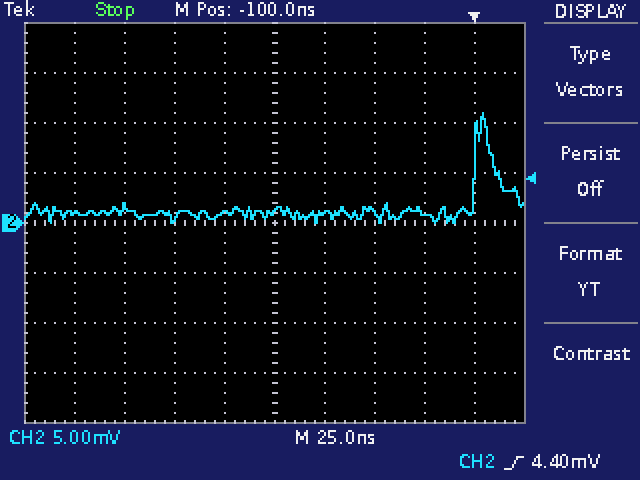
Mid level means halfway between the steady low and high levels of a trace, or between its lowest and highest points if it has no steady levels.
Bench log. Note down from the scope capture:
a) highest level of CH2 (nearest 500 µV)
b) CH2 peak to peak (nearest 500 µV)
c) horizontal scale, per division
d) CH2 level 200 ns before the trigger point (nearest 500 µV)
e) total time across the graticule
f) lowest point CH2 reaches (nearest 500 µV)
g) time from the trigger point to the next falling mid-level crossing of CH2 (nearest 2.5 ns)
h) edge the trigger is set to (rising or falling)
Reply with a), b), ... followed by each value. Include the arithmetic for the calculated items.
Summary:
a) 11.0 mV
b) 11.0 mV − (0.0 mV) = 11.0 mV
c) 25 ns
d) 1.0 mV
e) 250 ns
f) 0.0 mV
g) 10.0 ns
h) rising
